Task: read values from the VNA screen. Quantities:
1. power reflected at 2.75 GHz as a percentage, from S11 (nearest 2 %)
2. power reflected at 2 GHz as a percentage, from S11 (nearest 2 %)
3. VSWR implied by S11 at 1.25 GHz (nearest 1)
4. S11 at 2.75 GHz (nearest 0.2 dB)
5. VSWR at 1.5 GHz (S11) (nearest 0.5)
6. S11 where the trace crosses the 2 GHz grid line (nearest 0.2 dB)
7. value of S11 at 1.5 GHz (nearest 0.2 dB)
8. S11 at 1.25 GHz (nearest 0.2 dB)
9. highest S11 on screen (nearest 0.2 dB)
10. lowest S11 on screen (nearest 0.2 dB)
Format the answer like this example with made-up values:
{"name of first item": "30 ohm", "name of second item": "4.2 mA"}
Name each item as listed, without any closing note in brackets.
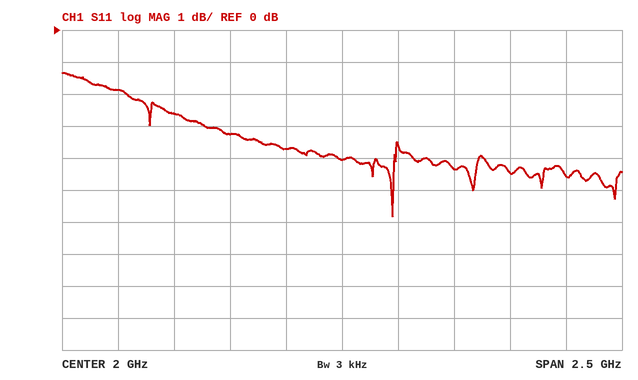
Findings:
{"power reflected at 2.75 GHz as a percentage, from S11": "36 %", "power reflected at 2 GHz as a percentage, from S11": "40 %", "VSWR implied by S11 at 1.25 GHz": "7", "S11 at 2.75 GHz": "-4.4 dB", "VSWR at 1.5 GHz (S11)": "5.5", "S11 where the trace crosses the 2 GHz grid line": "-4.0 dB", "value of S11 at 1.5 GHz": "-3.2 dB", "S11 at 1.25 GHz": "-2.6 dB", "highest S11 on screen": "-1.4 dB", "lowest S11 on screen": "-5.8 dB"}
